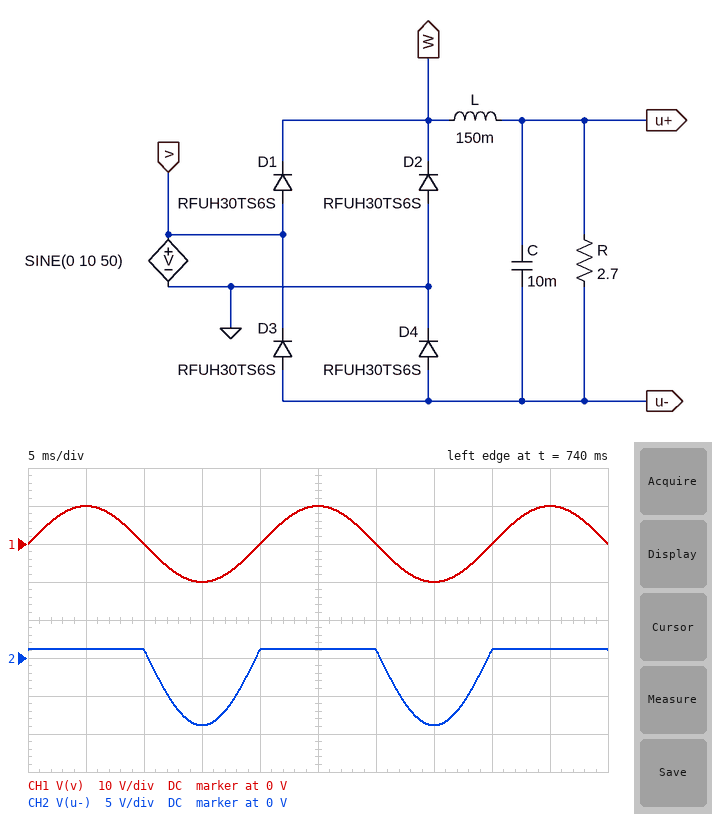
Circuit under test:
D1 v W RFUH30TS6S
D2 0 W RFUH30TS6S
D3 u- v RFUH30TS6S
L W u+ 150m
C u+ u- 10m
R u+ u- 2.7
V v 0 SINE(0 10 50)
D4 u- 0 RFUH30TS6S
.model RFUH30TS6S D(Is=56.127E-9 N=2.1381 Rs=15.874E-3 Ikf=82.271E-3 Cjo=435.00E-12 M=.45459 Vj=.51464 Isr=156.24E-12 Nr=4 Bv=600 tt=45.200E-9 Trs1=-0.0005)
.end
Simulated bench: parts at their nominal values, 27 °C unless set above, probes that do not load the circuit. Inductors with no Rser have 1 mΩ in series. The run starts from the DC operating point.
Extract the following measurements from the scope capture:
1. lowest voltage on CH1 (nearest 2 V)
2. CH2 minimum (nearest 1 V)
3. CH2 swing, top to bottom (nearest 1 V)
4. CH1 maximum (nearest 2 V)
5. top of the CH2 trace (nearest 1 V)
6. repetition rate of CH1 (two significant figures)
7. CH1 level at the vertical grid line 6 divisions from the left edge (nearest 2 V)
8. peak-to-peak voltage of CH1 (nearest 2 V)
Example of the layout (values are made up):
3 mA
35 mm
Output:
-10 V
-9 V
10 V
10 V
1 V
50 Hz
0 V
20 V
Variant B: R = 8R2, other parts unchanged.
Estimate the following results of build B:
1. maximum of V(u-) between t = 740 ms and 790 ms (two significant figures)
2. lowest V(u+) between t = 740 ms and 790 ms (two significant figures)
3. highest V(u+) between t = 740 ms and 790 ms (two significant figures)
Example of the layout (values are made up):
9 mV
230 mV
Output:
1.0 V
-4.7 V
5.4 V
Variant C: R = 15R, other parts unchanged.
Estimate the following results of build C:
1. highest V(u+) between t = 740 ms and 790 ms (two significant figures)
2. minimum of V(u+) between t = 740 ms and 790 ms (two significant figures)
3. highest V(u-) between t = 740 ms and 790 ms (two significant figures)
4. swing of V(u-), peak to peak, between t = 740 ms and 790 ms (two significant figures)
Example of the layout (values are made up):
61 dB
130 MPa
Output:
5.4 V
-4.6 V
970 mV
10 V
